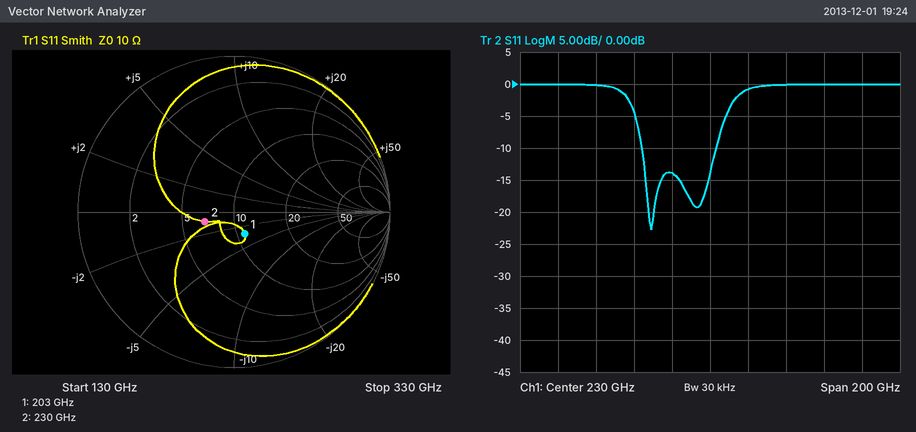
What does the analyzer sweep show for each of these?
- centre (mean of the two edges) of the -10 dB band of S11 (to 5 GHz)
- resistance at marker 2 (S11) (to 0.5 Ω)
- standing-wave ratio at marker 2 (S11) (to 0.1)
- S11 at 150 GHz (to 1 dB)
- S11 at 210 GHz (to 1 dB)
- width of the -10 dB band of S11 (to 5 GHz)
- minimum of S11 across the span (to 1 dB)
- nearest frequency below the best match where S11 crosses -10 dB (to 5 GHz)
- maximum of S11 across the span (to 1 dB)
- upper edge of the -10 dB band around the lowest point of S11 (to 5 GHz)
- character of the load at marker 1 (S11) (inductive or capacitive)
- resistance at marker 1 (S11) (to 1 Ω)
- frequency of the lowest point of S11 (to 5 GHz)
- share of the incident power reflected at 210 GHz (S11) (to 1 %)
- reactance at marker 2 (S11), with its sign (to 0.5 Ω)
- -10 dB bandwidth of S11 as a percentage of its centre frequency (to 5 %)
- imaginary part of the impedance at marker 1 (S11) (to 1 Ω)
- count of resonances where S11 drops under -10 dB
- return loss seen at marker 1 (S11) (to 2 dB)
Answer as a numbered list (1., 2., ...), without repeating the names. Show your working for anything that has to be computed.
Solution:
1. 215 GHz
2. 7.0 Ω
3. 1.5
4. 0 dB
5. -14 dB
6. 235 GHz − 195 GHz = 40 GHz
7. -23 dB
8. 195 GHz
9. 0 dB
10. 235 GHz
11. capacitive
12. 11 Ω
13. 200 GHz
14. 10^(-14/10) ≈ 4 %
15. -1.0 Ω
16. 40 GHz / 215 GHz ≈ 18.6 %, so 20 % to the nearest 5 %
17. -3 Ω
18. 2
19. 16 dB
